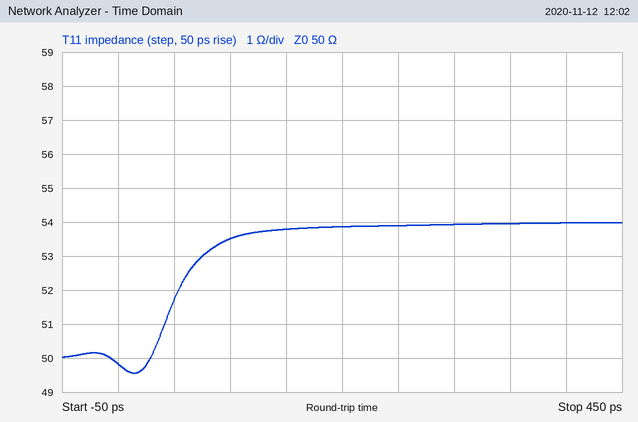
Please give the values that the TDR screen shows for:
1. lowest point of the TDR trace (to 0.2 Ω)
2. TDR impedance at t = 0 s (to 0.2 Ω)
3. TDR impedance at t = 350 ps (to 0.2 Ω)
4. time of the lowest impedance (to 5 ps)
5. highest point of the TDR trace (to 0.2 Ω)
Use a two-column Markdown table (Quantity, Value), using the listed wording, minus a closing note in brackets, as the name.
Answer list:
| Quantity | Value |
|---|---|
| lowest point of the TDR trace | 49.6 Ω |
| TDR impedance at t = 0 s | 49.8 Ω |
| TDR impedance at t = 350 ps | 54.0 Ω |
| time of the lowest impedance | 15 ps |
| highest point of the TDR trace | 54.0 Ω |
